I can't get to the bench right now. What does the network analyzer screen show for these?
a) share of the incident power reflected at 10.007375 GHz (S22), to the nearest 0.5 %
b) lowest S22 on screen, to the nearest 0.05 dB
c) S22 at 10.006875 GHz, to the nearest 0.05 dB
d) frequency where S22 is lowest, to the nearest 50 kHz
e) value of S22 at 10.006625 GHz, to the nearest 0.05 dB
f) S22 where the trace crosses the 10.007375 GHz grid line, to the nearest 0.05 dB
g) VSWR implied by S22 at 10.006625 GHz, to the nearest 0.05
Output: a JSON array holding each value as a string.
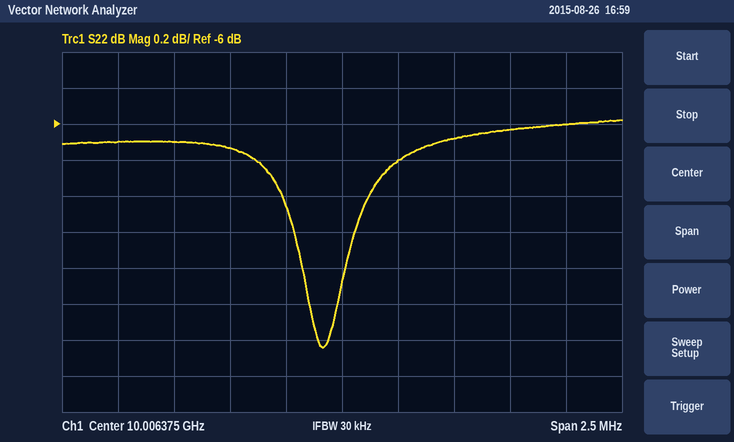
["25.0 %", "-7.25 dB", "-6.10 dB", "10.00630 GHz", "-6.20 dB", "-6.00 dB", "2.90"]
